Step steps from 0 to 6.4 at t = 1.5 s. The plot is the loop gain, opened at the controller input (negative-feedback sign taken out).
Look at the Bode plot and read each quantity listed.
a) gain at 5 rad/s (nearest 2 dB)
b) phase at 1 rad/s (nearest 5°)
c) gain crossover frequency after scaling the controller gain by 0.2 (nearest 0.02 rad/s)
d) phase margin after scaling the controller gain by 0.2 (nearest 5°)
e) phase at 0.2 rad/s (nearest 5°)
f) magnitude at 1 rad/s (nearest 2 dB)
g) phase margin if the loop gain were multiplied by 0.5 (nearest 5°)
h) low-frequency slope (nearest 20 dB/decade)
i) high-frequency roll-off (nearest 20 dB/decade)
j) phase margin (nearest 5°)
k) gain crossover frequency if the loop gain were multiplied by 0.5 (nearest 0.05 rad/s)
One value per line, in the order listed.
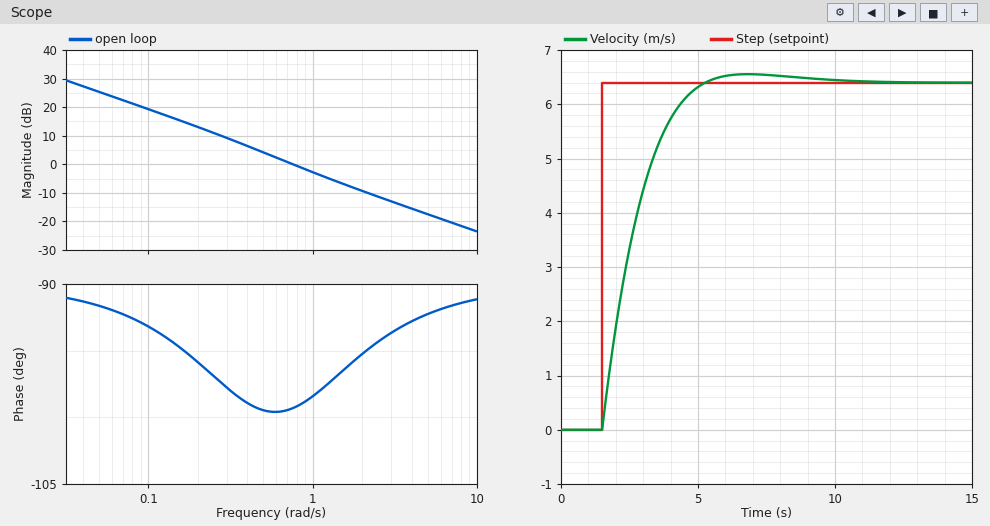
-18 dB
-100°
0.18 rad/s
85°
-95°
-2 dB
80°
-20 dB/decade
-20 dB/decade
80°
0.40 rad/s
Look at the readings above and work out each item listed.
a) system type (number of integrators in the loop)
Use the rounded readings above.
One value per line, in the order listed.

1
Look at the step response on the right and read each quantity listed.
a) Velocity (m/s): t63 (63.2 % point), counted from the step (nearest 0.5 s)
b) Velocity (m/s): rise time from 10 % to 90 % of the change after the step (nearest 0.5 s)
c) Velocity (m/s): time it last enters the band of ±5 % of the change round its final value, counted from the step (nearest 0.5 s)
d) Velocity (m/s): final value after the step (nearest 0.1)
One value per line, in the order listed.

1.5 s
2.5 s
3.0 s
6.4
